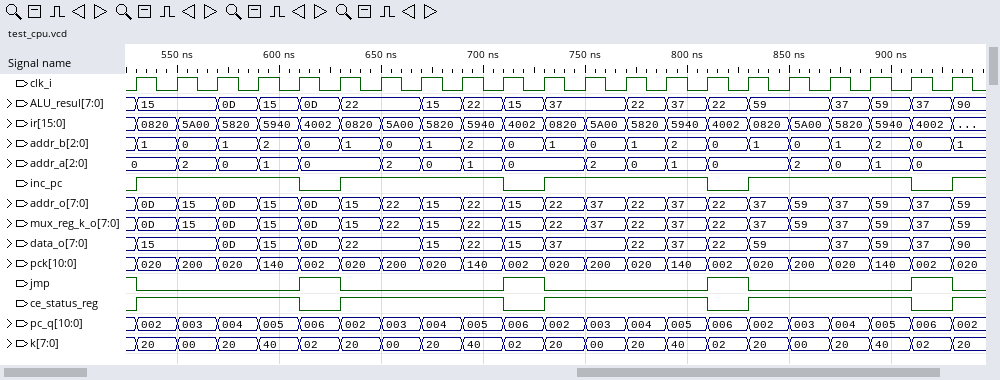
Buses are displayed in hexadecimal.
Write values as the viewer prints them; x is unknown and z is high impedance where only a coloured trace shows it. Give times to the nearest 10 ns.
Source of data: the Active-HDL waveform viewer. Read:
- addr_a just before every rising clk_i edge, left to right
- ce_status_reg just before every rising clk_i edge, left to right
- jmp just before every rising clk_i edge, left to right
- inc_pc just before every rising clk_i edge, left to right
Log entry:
0, 0, 2, 0, 1, 0, 0, 2, 0, 1, 0, 0, 2, 0, 1, 0, 0, 2, 0, 1, 0
0 1 1 1 1 0 1 1 1 1 0 1 1 1 1 0 1 1 1 1 0
1 0 0 0 0 1 0 0 0 0 1 0 0 0 0 1 0 0 0 0 1
0 1 1 1 1 0 1 1 1 1 0 1 1 1 1 0 1 1 1 1 0
